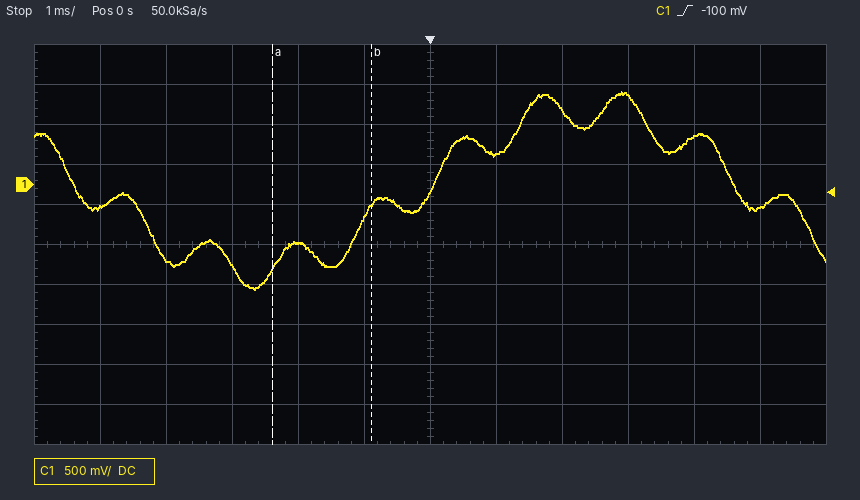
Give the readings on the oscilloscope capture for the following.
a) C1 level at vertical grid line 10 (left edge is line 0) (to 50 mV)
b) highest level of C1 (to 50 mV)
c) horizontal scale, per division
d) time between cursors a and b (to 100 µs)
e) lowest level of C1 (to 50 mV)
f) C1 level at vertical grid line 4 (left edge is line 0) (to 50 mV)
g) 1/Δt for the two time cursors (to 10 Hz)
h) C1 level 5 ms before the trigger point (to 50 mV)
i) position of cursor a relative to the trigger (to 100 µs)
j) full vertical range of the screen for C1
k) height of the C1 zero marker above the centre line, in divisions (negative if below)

600 mV
1.15 V
1 ms
1.5 ms
-1.30 V
-750 mV
670 Hz
-300 mV
-2.4 ms
5 V
+1.5 div
